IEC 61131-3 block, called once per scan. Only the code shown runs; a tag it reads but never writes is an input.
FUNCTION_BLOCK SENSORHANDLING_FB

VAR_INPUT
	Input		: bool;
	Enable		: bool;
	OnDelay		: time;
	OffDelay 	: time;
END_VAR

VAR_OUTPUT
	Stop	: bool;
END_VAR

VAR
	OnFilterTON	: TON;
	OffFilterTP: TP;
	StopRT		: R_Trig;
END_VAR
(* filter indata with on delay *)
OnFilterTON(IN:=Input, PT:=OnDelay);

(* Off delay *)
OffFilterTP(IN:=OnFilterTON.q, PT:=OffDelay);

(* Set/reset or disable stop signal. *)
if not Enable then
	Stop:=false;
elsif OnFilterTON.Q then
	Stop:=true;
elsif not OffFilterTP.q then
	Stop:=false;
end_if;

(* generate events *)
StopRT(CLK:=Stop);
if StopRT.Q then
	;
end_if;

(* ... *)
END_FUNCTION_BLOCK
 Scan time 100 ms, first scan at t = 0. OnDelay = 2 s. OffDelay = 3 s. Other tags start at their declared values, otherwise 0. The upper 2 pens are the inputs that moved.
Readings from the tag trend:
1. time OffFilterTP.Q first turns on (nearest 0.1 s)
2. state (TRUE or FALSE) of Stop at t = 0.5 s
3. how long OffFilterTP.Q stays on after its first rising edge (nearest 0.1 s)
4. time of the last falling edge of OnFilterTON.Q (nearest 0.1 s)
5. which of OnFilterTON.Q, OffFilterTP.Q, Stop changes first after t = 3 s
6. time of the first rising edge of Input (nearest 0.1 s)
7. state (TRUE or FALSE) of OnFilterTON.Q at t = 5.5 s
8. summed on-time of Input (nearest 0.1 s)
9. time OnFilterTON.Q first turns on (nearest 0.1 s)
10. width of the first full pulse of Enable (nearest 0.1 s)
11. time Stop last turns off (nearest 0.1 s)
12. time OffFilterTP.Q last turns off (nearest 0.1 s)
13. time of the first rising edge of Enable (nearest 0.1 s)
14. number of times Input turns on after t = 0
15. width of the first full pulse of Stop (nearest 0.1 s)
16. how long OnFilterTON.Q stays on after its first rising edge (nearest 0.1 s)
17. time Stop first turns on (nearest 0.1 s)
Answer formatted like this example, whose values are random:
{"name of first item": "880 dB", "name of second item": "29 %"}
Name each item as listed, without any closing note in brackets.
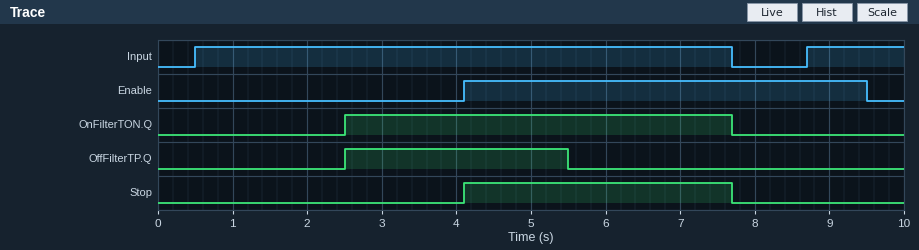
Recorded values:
{"time OffFilterTP.Q first turns on": "2.5 s", "state (TRUE or FALSE) of Stop at t = 0.5 s": "FALSE", "how long OffFilterTP.Q stays on after its first rising edge": "3.0 s", "time of the last falling edge of OnFilterTON.Q": "7.7 s", "which of OnFilterTON.Q, OffFilterTP.Q, Stop changes first after t = 3 s": "Stop", "time of the first rising edge of Input": "0.5 s", "state (TRUE or FALSE) of OnFilterTON.Q at t = 5.5 s": "TRUE", "summed on-time of Input": "8.5 s", "time OnFilterTON.Q first turns on": "2.5 s", "width of the first full pulse of Enable": "5.4 s", "time Stop last turns off": "7.7 s", "time OffFilterTP.Q last turns off": "5.5 s", "time of the first rising edge of Enable": "4.1 s", "number of times Input turns on after t = 0": "2", "width of the first full pulse of Stop": "3.6 s", "how long OnFilterTON.Q stays on after its first rising edge": "5.2 s", "time Stop first turns on": "4.1 s"}
